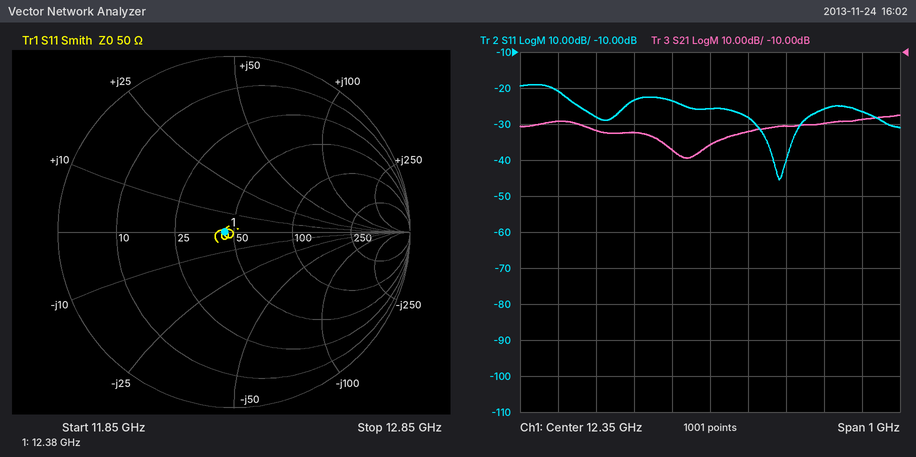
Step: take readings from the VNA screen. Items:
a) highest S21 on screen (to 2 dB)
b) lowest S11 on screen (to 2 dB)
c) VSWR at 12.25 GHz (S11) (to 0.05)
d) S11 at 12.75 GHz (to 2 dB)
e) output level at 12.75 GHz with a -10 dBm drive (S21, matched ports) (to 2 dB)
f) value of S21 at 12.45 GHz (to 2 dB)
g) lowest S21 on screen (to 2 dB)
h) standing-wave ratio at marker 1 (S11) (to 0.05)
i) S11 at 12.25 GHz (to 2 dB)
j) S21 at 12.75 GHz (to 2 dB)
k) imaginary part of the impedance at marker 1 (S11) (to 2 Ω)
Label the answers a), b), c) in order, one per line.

a) -28 dB
b) -46 dB
c) 1.15
d) -26 dB
e) -38 dBm
f) -32 dB
g) -40 dB
h) 1.10
i) -24 dB
j) -28 dB
k) 0 Ω
